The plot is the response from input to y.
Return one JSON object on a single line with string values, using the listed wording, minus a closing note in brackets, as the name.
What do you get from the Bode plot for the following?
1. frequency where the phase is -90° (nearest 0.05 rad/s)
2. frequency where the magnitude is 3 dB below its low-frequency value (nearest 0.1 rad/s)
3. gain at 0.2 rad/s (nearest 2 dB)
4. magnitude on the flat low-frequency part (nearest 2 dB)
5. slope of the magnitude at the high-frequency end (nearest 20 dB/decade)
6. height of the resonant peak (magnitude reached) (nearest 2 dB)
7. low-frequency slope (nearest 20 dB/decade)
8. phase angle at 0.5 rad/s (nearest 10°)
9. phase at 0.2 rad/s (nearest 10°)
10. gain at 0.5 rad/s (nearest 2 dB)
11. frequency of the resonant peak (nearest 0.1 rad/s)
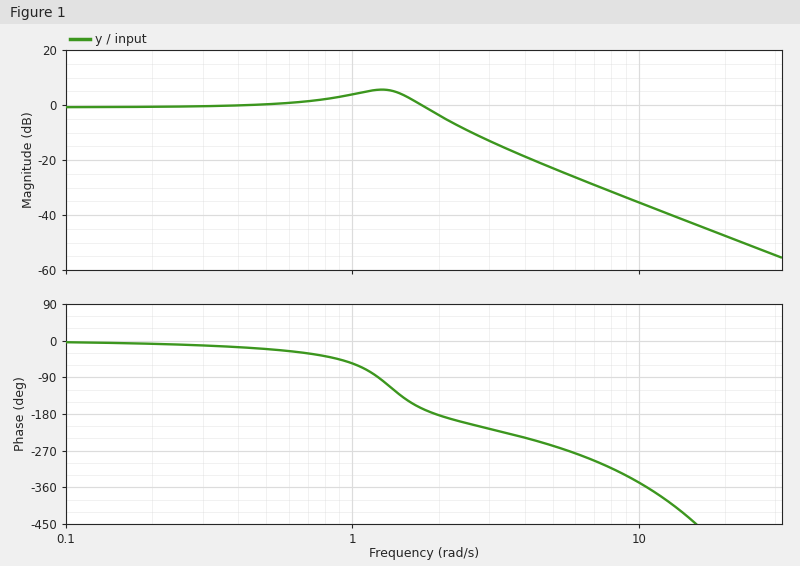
{"frequency where the phase is -90°": "1.25 rad/s", "frequency where the magnitude is 3 dB below its low-frequency value": "2.0 rad/s", "gain at 0.2 rad/s": "0 dB", "magnitude on the flat low-frequency part": "0 dB", "slope of the magnitude at the high-frequency end": "-40 dB/decade", "height of the resonant peak (magnitude reached)": "6 dB", "low-frequency slope": "0 dB/decade", "phase angle at 0.5 rad/s": "-20°", "phase at 0.2 rad/s": "-10°", "gain at 0.5 rad/s": "0 dB", "frequency of the resonant peak": "1.3 rad/s"}
